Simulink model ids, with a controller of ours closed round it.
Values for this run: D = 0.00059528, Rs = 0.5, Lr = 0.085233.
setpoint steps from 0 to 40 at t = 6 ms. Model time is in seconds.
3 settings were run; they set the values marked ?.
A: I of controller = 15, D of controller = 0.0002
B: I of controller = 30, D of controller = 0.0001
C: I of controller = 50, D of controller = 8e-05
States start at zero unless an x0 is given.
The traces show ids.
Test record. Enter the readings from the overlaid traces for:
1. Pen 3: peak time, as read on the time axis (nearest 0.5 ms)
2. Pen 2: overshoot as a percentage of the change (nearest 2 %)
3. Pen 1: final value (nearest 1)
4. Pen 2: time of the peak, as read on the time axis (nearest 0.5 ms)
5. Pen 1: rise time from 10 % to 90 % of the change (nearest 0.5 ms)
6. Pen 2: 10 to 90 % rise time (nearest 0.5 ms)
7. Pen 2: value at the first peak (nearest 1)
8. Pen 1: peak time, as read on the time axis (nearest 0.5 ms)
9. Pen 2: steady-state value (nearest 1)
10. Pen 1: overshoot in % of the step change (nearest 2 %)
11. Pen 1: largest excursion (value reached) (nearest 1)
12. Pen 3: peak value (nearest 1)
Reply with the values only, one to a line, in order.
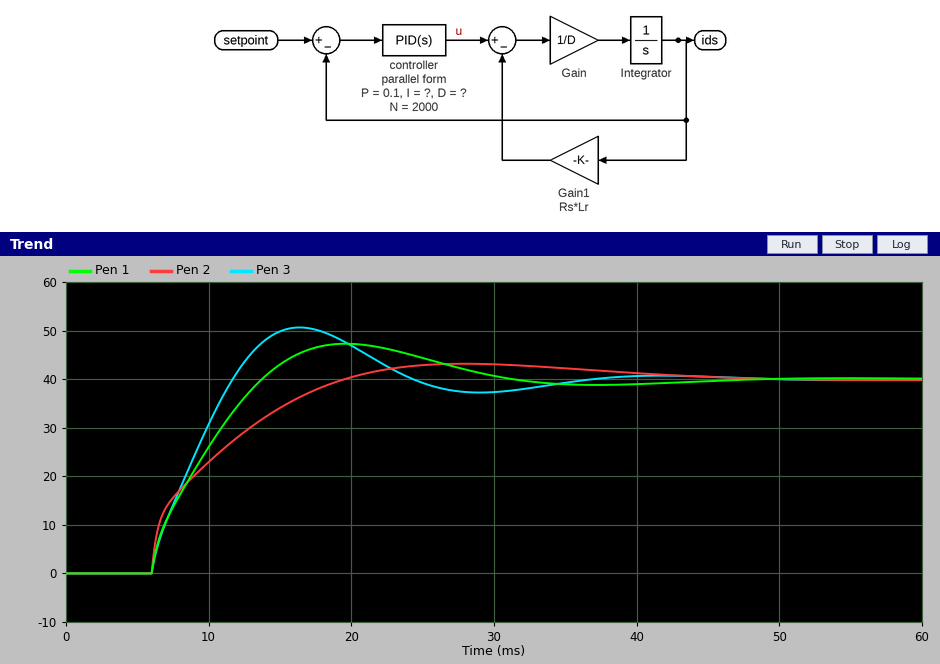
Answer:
16.5 ms
8 %
40
28.0 ms
6.0 ms
10.0 ms
43
19.5 ms
40
18 %
47
51
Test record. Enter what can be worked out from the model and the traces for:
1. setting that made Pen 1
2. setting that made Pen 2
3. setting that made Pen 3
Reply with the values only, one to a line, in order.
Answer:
B
A
C
